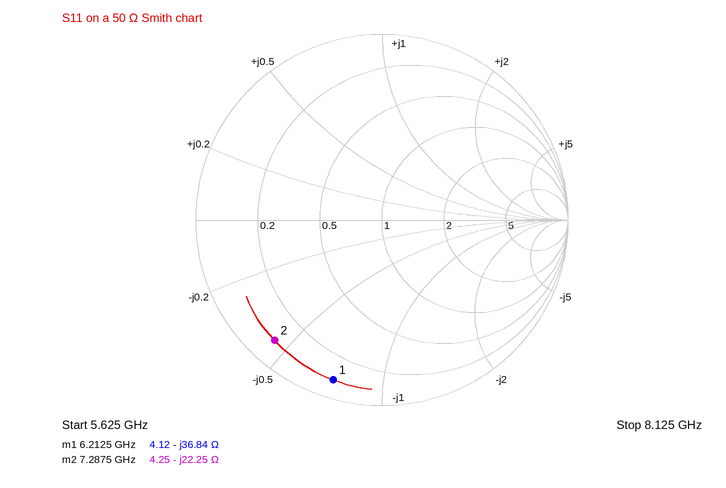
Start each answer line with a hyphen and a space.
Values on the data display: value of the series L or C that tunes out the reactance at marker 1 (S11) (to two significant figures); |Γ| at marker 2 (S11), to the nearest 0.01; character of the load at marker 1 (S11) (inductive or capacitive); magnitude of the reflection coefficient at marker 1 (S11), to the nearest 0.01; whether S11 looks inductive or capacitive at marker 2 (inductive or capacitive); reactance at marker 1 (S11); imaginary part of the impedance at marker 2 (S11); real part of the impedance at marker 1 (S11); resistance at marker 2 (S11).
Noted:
- 940 pH
- 0.87
- capacitive
- 0.90
- capacitive
- -36.84 Ω
- -22.25 Ω
- 4.12 Ω
- 4.25 Ω
